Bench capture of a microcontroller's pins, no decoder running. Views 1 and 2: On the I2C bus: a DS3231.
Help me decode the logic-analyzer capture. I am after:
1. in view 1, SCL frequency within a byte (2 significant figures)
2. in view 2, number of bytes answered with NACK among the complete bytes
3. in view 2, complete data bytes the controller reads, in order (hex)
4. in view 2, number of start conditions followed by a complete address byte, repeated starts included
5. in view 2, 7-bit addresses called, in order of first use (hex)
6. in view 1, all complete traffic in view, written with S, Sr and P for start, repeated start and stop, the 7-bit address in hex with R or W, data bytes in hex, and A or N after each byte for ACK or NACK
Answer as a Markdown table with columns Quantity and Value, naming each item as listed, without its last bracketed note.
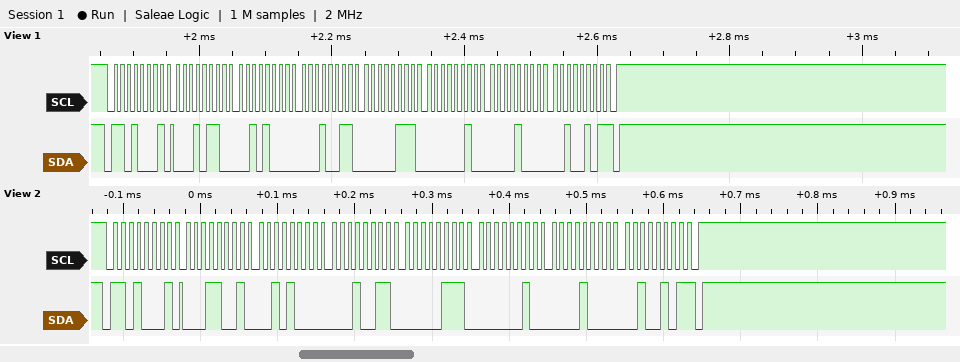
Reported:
| Quantity | Value |
|---|---|
| in view 1, SCL frequency within a byte | 100 kHz |
| in view 2, number of bytes answered with NACK among the complete bytes | 1 |
| in view 2, complete data bytes the controller reads, in order | 19 28 13 07 02 08 25 |
| in view 2, number of start conditions followed by a complete address byte, repeated starts included | 1 |
| in view 2, 7-bit addresses called, in order of first use | 0x68 |
| in view 1, all complete traffic in view, written with S, Sr and P for start, repeated start and stop, the 7-bit address in hex with R or W, data bytes in hex, and A or N after each byte for ACK or NACK | S 68R A 16 A 28 A 13 A 07 A 02 A 08 A 25 N P |
